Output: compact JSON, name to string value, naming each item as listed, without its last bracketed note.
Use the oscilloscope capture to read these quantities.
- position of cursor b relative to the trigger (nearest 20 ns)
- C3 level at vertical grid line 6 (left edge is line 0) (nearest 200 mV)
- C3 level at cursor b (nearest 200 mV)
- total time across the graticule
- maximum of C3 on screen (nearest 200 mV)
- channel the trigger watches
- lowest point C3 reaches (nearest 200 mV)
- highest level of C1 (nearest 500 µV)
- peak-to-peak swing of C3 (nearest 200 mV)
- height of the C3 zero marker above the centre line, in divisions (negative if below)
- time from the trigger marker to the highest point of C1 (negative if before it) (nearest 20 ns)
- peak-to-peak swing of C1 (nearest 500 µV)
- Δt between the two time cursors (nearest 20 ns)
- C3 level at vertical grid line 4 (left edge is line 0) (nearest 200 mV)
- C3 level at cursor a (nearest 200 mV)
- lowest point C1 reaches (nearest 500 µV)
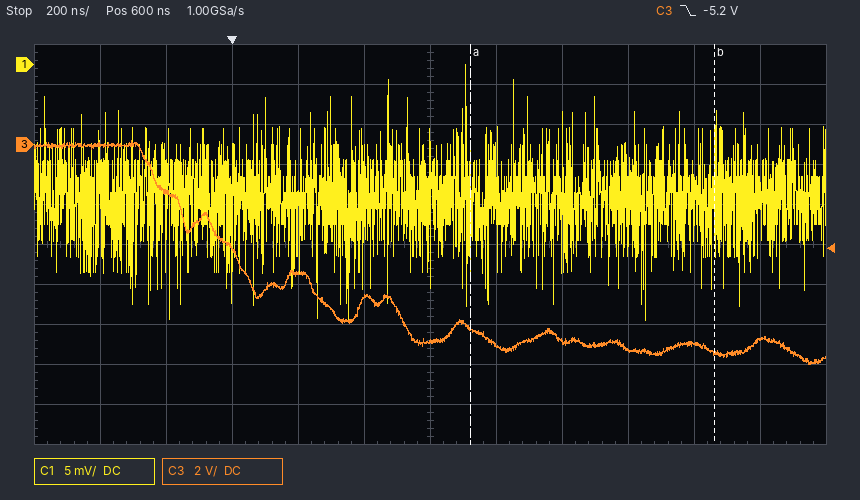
{"position of cursor b relative to the trigger": "+1.46 µs", "C3 level at vertical grid line 6 (left edge is line 0)": "-9.8 V", "C3 level at cursor b": "-10.4 V", "total time across the graticule": "2.4 µs", "maximum of C3 on screen": "200 mV", "channel the trigger watches": "C3", "lowest point C3 reaches": "-11.0 V", "highest level of C1": "0.0 mV", "peak-to-peak swing of C3": "11.2 V", "height of the C3 zero marker above the centre line, in divisions": "+2.5 div", "time from the trigger marker to the highest point of C1 (negative if before it)": "+700 ns", "peak-to-peak swing of C1": "32.0 mV", "Δt between the two time cursors": "740 ns", "C3 level at vertical grid line 4 (left edge is line 0)": "-6.4 V", "C3 level at cursor a": "-9.2 V", "lowest point C1 reaches": "-32.0 mV"}
